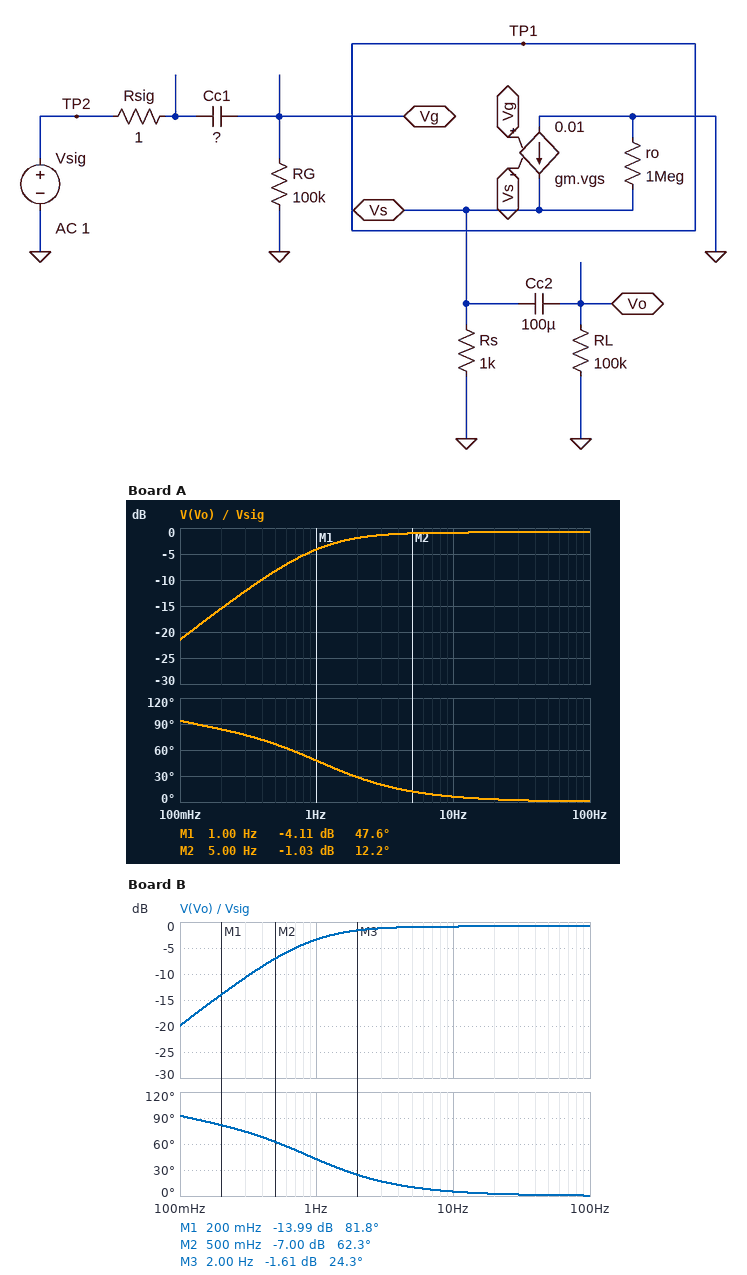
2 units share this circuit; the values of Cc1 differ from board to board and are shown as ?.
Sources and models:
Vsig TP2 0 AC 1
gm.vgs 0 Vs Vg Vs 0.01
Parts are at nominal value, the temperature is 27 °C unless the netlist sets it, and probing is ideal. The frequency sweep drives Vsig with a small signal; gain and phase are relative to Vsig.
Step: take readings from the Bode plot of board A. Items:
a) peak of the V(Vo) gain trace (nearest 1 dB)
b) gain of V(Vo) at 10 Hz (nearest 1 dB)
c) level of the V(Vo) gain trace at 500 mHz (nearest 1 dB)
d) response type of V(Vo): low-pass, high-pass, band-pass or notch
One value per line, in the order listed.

-1 dB
-1 dB
-8 dB
high-pass
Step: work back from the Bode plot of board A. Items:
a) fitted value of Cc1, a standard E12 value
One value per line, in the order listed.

1.5 µF
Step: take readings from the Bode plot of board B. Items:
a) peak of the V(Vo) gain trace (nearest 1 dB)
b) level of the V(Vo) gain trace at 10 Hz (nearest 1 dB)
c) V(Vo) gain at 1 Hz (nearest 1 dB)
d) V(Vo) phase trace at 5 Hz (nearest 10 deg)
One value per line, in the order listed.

-1 dB
-1 dB
-3 dB
10 deg
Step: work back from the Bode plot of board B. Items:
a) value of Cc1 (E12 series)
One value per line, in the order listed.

1.8 µF
